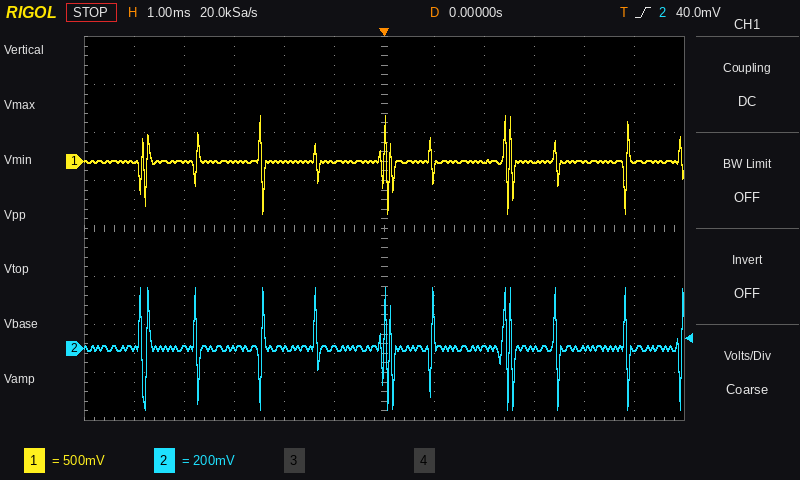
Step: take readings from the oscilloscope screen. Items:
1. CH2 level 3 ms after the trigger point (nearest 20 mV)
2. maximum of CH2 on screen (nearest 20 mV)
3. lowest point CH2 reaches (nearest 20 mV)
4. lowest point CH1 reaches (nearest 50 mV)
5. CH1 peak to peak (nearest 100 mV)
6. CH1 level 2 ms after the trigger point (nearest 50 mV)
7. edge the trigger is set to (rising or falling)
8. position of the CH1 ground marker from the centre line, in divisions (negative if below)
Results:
0 mV
260 mV
-260 mV
-550 mV
1.00 V
0 mV
rising
+1.4 div
